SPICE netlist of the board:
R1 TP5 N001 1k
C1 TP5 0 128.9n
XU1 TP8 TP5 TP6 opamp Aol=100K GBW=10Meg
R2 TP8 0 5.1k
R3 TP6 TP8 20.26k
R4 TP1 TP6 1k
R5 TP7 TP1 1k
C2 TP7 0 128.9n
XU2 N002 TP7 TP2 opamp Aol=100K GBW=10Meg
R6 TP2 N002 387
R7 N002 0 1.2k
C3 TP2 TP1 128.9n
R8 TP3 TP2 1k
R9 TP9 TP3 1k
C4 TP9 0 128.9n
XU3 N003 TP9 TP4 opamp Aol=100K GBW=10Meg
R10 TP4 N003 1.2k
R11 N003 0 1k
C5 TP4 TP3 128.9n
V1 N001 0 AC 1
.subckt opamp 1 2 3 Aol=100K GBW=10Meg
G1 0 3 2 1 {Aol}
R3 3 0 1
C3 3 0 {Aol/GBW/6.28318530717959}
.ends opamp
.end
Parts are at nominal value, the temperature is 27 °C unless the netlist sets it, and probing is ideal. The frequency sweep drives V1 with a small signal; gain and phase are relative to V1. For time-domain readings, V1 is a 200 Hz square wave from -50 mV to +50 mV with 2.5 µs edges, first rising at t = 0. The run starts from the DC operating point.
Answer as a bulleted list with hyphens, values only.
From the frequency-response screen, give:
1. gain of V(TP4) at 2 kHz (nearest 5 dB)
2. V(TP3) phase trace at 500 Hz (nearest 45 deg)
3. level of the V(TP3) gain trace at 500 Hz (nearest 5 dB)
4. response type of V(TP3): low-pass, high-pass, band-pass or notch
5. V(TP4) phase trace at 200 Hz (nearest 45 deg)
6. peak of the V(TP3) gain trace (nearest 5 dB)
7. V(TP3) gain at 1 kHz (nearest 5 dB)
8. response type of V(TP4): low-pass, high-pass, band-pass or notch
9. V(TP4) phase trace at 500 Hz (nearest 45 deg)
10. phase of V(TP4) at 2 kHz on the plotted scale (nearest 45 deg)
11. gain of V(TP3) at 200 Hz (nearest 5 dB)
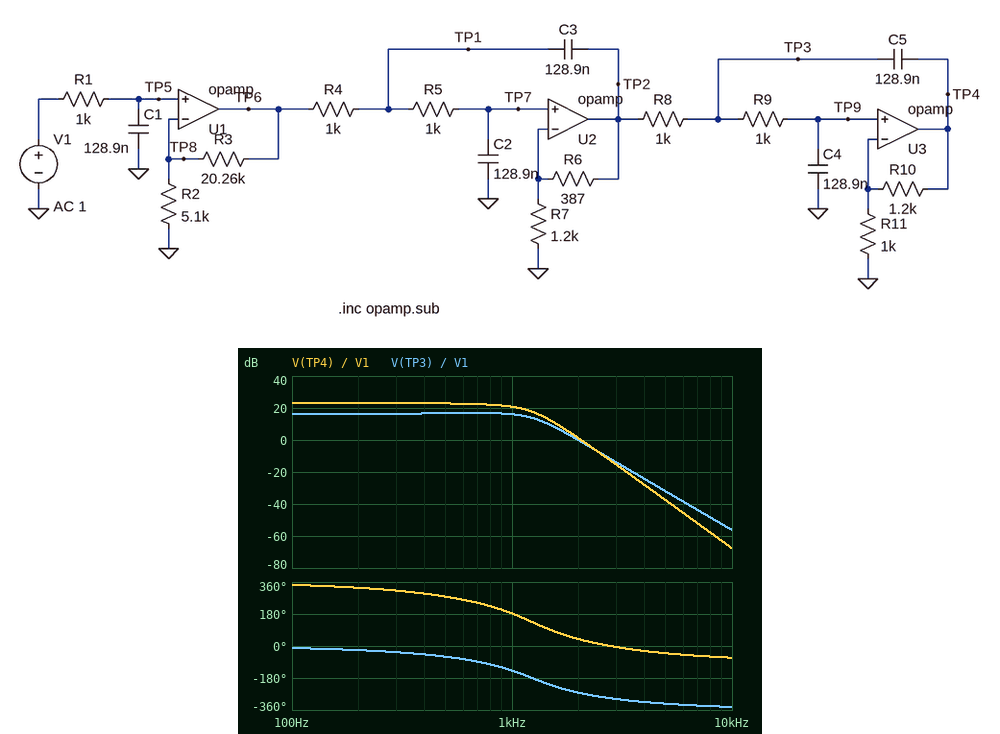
- 0 dB
- -45 deg
- 15 dB
- low-pass
- 315 deg
- 15 dB
- 15 dB
- low-pass
- 270 deg
- 45 deg
- 15 dB
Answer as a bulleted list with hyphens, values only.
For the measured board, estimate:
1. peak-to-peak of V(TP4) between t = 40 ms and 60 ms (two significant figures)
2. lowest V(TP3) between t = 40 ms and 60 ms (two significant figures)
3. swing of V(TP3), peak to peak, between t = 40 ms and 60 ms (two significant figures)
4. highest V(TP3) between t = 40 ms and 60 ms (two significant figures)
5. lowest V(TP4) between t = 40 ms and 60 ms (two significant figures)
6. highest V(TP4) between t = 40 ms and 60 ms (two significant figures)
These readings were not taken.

- 1.7 V
- -420 mV
- 840 mV
- 420 mV
- -830 mV
- 830 mV
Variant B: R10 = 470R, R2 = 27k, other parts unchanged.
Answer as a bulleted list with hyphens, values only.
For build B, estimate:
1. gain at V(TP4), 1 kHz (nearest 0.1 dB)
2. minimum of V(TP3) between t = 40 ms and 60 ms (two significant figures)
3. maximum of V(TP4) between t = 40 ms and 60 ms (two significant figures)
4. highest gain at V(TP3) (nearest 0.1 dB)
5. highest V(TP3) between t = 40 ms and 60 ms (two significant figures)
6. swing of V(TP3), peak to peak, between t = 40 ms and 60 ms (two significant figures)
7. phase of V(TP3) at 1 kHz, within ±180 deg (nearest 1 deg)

- 3.3 dB
- -120 mV
- 170 mV
- 7.3 dB
- 120 mV
- 240 mV
- -150 deg
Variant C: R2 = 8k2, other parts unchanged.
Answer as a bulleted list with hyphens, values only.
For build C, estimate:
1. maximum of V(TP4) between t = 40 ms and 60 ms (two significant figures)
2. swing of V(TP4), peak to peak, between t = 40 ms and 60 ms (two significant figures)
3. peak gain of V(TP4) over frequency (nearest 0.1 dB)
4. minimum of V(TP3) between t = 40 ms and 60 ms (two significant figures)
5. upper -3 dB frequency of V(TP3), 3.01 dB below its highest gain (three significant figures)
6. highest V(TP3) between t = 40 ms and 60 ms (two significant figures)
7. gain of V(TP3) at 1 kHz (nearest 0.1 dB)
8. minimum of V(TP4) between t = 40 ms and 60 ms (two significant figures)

- 580 mV
- 1.2 V
- 20.1 dB
- -290 mV
- 1.24 kHz
- 290 mV
- 13.0 dB
- -580 mV
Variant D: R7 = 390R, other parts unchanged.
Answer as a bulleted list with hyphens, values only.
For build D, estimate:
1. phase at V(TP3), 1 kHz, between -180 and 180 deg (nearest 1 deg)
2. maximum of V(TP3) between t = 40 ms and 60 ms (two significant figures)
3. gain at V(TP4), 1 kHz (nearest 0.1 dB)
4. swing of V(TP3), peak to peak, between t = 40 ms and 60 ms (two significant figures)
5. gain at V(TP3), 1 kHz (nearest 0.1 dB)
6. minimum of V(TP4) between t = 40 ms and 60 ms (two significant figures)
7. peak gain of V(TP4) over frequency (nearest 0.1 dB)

- -129 deg
- 850 mV
- 28.3 dB
- 1.7 V
- 23.7 dB
- -1.6 V
- 28.7 dB
